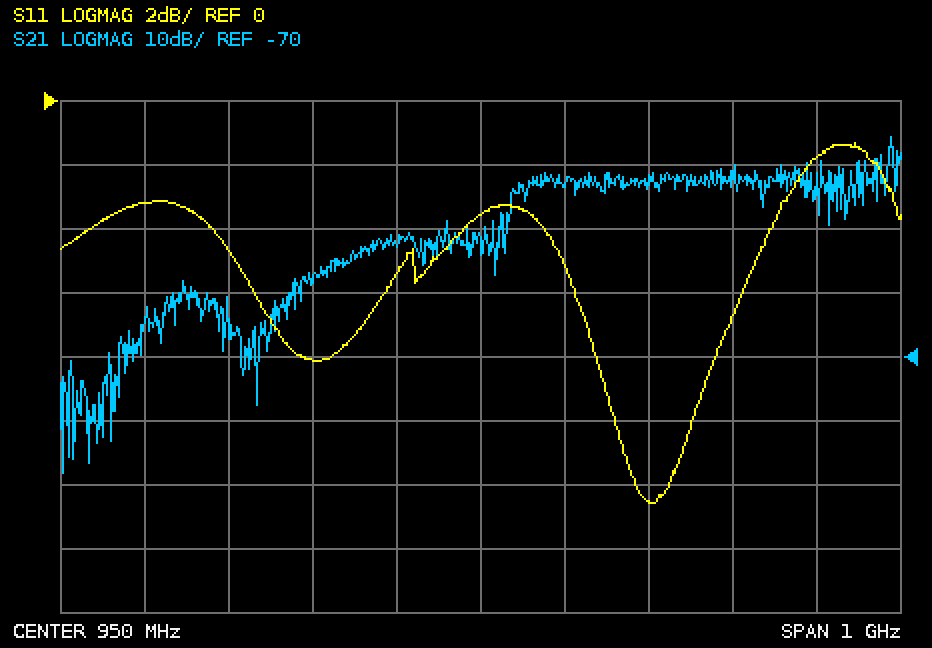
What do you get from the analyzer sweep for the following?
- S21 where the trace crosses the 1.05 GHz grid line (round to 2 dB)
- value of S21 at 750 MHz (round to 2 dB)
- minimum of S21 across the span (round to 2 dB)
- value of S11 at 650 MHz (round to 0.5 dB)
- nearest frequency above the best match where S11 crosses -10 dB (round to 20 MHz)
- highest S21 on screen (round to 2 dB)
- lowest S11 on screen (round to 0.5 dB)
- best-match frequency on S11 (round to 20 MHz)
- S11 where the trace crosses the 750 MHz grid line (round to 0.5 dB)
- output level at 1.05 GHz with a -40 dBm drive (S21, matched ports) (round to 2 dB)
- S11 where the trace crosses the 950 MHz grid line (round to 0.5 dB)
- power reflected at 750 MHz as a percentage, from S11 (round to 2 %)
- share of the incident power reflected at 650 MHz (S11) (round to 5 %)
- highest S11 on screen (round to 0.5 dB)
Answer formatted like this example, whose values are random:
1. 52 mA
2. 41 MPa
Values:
1. -44 dB
2. -58 dB
3. -88 dB
4. -4.5 dB
5. 1.20 GHz
6. -36 dB
7. -12.5 dB
8. 1.16 GHz
9. -8.0 dB
10. -84 dBm
11. -3.5 dB
12. 16 %
13. 35 %
14. -1.5 dB
